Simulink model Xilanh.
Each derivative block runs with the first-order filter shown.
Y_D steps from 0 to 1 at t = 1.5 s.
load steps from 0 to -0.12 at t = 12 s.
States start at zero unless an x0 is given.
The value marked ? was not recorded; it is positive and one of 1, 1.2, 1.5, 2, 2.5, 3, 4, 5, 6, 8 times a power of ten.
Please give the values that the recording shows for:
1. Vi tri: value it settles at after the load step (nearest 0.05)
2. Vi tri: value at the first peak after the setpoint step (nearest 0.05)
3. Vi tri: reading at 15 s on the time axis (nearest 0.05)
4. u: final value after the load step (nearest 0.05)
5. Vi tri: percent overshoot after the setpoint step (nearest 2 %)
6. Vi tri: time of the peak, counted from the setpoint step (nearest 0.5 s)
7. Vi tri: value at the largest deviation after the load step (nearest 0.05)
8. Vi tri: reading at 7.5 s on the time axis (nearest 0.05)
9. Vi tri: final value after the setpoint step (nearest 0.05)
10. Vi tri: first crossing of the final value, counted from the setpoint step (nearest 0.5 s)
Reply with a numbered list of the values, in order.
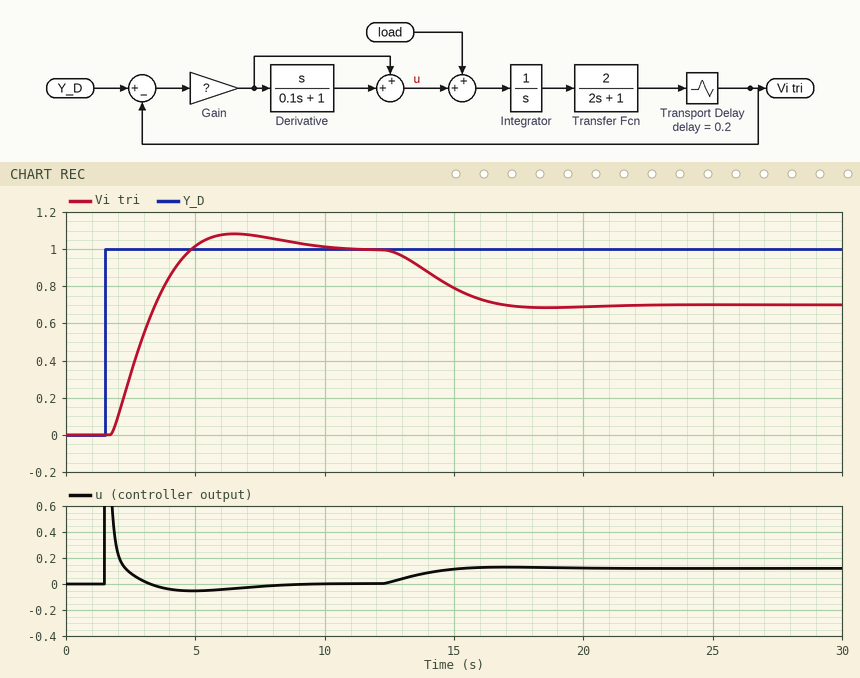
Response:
1. 0.70
2. 1.10
3. 0.80
4. 0.10
5. 8 %
6. 5.0 s
7. 0.70
8. 1.05
9. 1.00
10. 3.5 s
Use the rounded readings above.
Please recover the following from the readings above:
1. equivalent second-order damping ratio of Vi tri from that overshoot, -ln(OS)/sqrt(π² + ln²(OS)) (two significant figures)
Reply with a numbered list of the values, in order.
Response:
1. 0.63
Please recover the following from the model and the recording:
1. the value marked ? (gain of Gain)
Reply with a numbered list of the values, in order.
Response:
1. 0.4
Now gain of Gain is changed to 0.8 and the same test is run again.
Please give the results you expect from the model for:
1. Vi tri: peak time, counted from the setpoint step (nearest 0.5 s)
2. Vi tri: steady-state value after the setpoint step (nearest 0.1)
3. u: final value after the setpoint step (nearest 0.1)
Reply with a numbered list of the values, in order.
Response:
1. 3.0 s
2. 1.0
3. 0.0
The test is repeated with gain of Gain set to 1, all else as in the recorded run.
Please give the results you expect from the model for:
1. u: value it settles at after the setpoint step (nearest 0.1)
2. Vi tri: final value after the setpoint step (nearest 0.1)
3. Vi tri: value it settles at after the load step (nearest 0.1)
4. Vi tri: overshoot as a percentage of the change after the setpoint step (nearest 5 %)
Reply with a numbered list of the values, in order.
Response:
1. 0.0
2. 1.0
3. 0.9
4. 15 %
